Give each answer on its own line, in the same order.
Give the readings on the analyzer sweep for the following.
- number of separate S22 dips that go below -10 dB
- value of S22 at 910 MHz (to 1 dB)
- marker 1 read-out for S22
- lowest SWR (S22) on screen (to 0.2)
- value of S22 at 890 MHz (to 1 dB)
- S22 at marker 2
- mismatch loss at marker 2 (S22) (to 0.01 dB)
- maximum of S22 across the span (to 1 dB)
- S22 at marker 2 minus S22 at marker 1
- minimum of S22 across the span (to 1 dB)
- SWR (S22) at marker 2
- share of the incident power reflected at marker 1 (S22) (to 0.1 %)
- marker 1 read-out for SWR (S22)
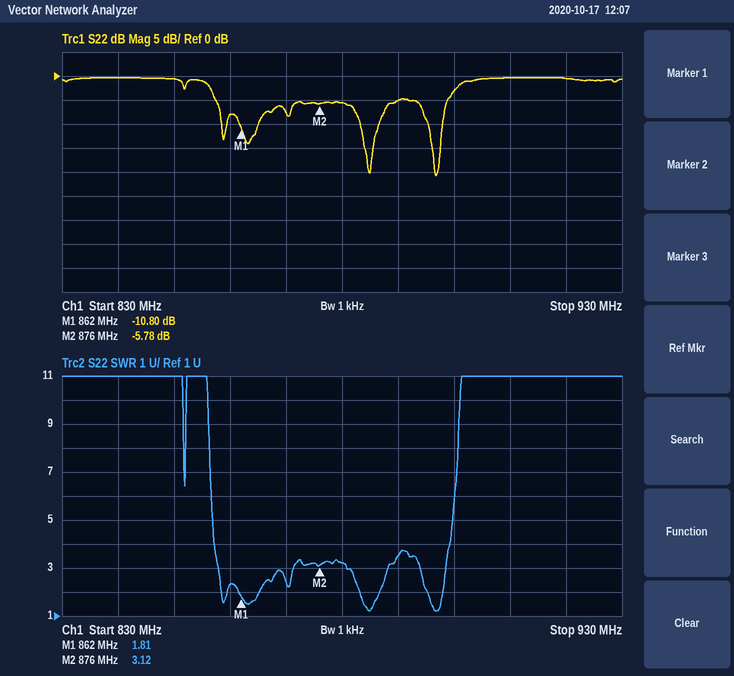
4
0 dB
-10.80 dB
1.2
-5 dB
-5.78 dB
1.33 dB
0 dB
5.02 dB
-21 dB
3.12
8.3 %
1.81
